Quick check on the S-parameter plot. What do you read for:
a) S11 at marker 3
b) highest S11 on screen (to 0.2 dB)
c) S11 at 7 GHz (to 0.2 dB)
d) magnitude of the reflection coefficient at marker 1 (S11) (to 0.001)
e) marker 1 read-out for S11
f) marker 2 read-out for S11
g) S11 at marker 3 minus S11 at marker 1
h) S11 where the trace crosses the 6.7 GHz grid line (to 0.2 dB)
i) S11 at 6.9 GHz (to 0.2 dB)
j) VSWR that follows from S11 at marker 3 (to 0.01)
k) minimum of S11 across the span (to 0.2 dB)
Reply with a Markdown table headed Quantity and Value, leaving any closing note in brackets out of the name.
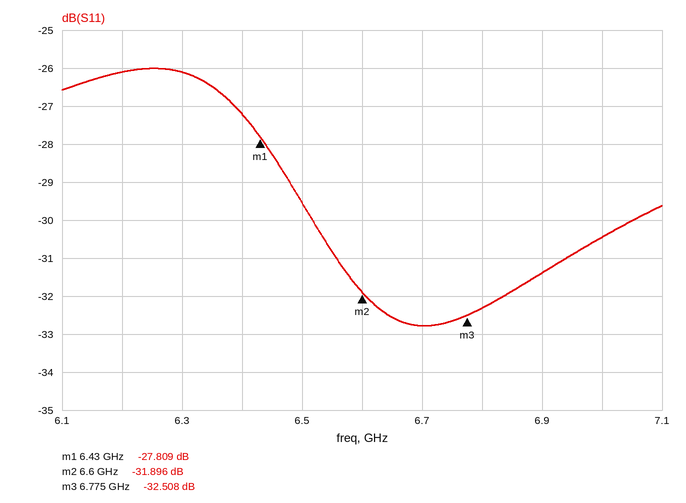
| Quantity | Value |
|---|---|
| S11 at marker 3 | -32.508 dB |
| highest S11 on screen | -26.0 dB |
| S11 at 7 GHz | -30.4 dB |
| magnitude of the reflection coefficient at marker 1 (S11) | 0.041 |
| marker 1 read-out for S11 | -27.809 dB |
| marker 2 read-out for S11 | -31.896 dB |
| S11 at marker 3 minus S11 at marker 1 | -4.699 dB |
| S11 where the trace crosses the 6.7 GHz grid line | -32.8 dB |
| S11 at 6.9 GHz | -31.4 dB |
| VSWR that follows from S11 at marker 3 | 1.05 |
| minimum of S11 across the span | -32.8 dB |
